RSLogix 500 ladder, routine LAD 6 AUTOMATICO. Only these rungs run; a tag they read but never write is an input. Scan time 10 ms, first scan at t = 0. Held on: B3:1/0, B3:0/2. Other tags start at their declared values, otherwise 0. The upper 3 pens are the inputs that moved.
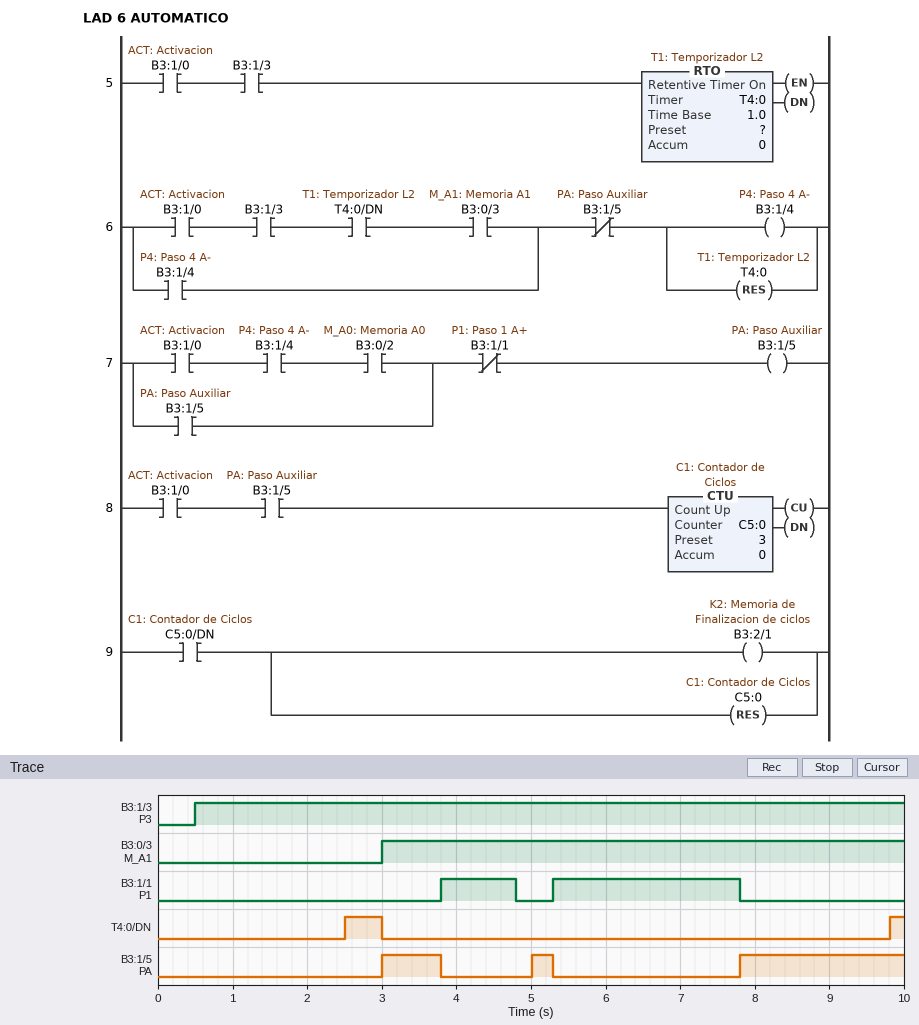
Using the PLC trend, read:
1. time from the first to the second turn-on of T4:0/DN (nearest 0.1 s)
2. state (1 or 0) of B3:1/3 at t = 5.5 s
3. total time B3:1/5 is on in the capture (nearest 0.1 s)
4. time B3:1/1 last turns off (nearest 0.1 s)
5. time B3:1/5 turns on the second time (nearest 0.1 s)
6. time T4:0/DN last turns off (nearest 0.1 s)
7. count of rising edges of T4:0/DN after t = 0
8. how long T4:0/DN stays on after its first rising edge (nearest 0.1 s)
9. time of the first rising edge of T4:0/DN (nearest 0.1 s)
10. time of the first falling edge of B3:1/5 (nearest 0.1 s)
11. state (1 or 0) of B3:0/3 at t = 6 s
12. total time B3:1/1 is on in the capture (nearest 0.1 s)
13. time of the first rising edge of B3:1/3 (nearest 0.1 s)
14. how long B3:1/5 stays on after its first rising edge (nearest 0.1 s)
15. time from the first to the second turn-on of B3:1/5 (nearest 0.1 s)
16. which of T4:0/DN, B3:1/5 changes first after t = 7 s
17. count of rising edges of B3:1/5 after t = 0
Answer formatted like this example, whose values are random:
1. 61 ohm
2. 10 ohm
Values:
1. 7.3 s
2. 1
3. 3.3 s
4. 7.8 s
5. 5.0 s
6. 3.0 s
7. 2
8. 0.5 s
9. 2.5 s
10. 3.8 s
11. 1
12. 3.5 s
13. 0.5 s
14. 0.8 s
15. 2.0 s
16. B3:1/5
17. 3
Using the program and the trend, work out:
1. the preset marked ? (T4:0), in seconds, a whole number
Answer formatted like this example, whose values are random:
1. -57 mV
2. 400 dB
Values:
1. 2 s
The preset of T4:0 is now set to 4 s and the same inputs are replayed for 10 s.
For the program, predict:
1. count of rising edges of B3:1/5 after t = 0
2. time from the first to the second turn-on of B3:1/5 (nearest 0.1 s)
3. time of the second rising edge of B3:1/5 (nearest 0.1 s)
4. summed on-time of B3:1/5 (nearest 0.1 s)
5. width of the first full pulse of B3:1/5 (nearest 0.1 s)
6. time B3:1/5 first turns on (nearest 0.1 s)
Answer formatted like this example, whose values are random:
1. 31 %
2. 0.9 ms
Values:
1. 2
2. 4.0 s
3. 8.8 s
4. 1.7 s
5. 0.5 s
6. 4.8 s
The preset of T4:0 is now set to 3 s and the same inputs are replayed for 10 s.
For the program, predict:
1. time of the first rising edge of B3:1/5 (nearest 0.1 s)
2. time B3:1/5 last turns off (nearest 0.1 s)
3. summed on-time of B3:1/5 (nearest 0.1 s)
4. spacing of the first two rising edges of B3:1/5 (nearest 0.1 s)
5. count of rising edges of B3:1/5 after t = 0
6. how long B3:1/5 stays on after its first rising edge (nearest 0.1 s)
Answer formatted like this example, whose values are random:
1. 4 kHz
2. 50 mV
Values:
1. 3.5 s
2. 3.8 s
3. 2.5 s
4. 4.3 s
5. 2
6. 0.3 s
